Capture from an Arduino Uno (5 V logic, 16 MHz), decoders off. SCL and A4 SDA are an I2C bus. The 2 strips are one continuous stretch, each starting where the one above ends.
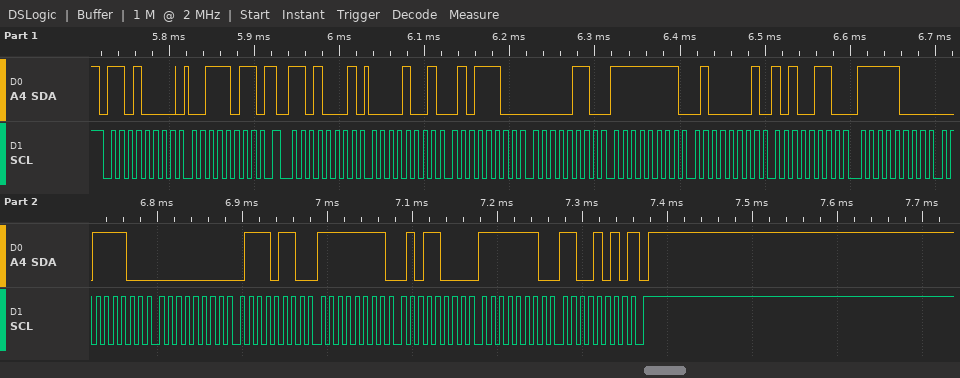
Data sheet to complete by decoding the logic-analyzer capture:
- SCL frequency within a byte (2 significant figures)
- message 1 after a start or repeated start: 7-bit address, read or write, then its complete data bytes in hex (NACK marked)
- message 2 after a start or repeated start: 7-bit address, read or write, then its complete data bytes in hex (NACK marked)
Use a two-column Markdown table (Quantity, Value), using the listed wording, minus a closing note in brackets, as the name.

| Quantity | Value |
|---|---|
| SCL frequency within a byte | 100 kHz |
| message 1 after a start or repeated start: 7-bit address, read or write, then its complete data bytes in hex | 0x68 write: 3B |
| message 2 after a start or repeated start: 7-bit address, read or write, then its complete data bytes in hex | 0x68 read: 09 5C 06 FF 41 A6 F8 3C 00 76 FF 58 FE CA NACK |
